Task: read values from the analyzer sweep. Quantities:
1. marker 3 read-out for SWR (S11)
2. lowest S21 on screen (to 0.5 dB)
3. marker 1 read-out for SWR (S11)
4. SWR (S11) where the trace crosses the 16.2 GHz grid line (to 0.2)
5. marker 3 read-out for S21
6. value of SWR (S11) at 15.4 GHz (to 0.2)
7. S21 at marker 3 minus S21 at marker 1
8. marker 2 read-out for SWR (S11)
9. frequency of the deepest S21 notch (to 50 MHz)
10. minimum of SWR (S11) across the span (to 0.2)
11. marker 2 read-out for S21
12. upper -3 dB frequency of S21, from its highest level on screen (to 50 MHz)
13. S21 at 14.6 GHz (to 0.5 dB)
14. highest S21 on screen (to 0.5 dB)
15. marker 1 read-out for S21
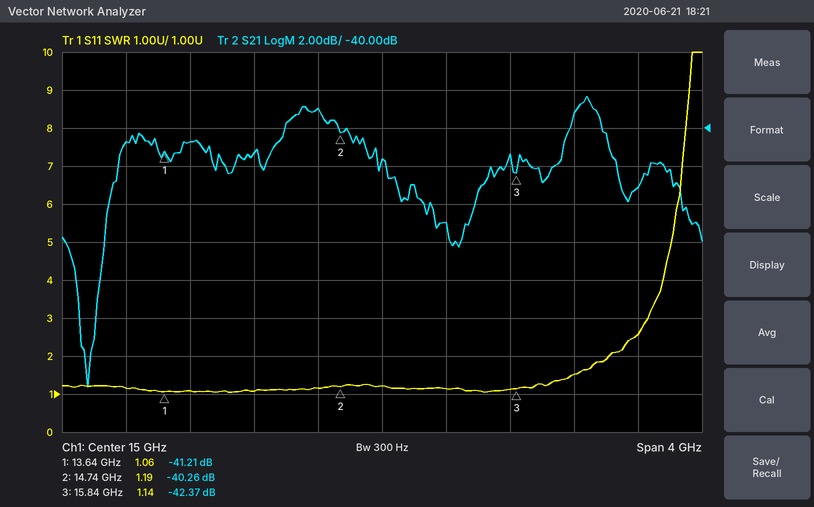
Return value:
1.14
-53.5 dB
1.06
1.6
-42.37 dB
1.2
-1.16 dB
1.19
13.15 GHz
1.0
-40.26 dB
16.45 GHz
-39.0 dB
-38.5 dB
-41.21 dB
